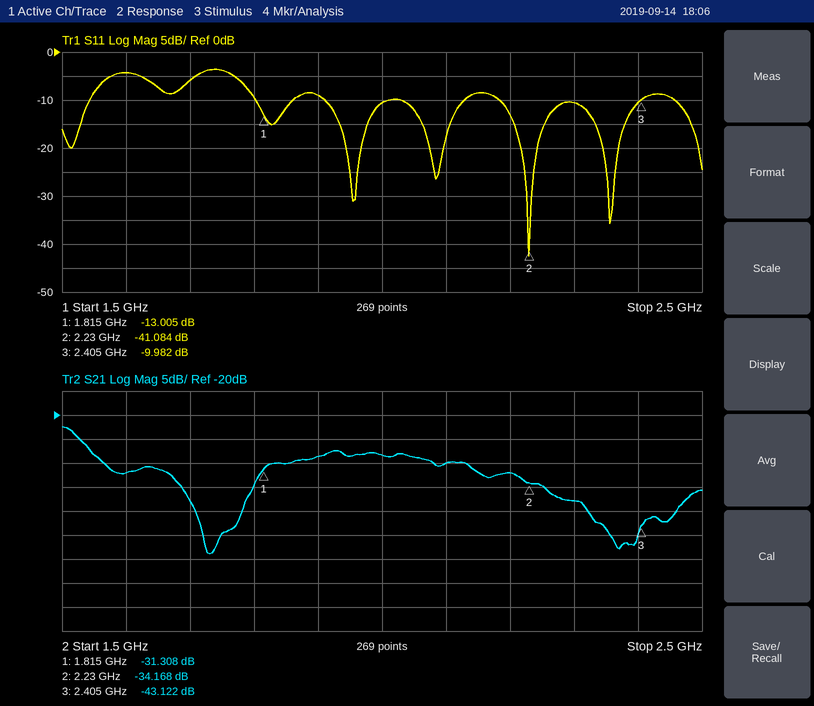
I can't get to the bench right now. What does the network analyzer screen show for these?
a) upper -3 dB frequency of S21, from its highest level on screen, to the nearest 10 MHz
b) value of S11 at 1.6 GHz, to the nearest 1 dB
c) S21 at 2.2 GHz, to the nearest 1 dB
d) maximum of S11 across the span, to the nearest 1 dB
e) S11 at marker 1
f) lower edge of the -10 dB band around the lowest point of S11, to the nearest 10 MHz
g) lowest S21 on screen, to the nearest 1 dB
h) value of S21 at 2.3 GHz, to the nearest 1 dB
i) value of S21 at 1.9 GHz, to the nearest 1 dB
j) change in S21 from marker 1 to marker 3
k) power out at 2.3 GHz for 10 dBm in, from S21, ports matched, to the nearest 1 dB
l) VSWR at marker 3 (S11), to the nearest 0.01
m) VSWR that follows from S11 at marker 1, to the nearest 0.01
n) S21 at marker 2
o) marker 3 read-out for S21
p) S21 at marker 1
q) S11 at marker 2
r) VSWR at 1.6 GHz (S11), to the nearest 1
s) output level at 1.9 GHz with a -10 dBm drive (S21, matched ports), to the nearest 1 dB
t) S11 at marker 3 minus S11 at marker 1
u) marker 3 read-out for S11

1.53 GHz
-4 dB
-32 dB
-4 dB
-13.005 dB
2.18 GHz
-49 dB
-38 dB
-29 dB
-11.814 dB
-28 dBm
1.93
1.58
-34.168 dB
-43.122 dB
-31.308 dB
-41.084 dB
4
-39 dBm
3.023 dB
-9.982 dB
